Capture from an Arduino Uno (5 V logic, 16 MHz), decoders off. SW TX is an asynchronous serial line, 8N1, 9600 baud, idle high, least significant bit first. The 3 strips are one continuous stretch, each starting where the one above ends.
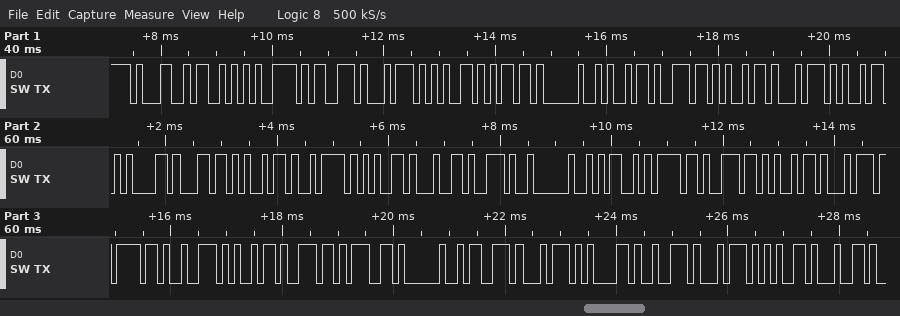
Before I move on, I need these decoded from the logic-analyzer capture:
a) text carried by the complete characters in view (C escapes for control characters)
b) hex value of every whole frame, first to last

"1System initialized. Monitoring started"
31 53 79 73 74 65 6D 20 69 6E 69 74 69 61 6C 69 7A 65 64 2E 20 4D 6F 6E 69 74 6F 72 69 6E 67 20 73 74 61 72 74 65 64
